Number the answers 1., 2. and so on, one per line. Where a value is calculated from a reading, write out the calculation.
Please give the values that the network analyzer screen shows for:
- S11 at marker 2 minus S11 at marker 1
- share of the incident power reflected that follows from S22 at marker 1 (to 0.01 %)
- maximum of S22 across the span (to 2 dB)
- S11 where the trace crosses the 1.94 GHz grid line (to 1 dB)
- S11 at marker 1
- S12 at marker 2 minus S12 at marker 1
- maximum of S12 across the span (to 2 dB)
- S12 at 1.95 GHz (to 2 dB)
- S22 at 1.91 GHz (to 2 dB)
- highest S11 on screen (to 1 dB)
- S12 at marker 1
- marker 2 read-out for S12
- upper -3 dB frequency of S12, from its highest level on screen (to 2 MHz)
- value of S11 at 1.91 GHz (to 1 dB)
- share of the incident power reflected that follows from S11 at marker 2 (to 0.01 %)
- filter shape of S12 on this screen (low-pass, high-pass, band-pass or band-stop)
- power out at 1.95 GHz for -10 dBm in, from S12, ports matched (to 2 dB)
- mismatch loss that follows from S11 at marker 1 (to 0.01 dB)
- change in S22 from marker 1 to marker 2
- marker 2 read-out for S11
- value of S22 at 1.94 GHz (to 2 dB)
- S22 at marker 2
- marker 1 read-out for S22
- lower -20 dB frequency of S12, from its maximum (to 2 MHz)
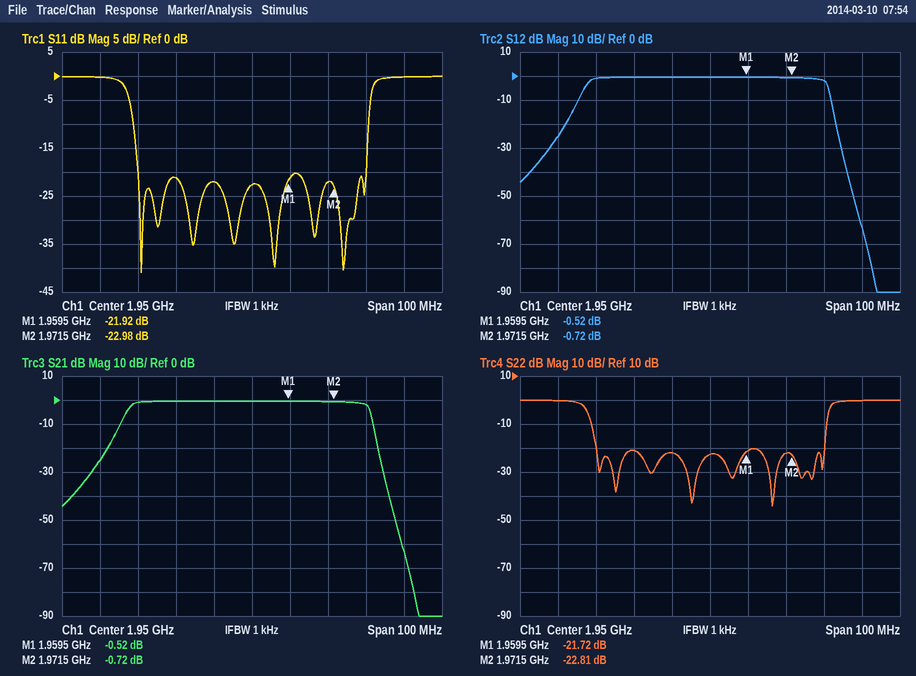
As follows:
1. -22.98 − (-21.92) = -1.06 dB
2. 10^(-21.72/10) ≈ 0.67 %
3. 0 dB
4. -22 dB
5. -21.92 dB
6. -0.72 − (-0.52) = -0.20 dB
7. 0 dB
8. 0 dB
9. 0 dB
10. 0 dB
11. -0.52 dB
12. -0.72 dB
13. 1.980 GHz
14. 0 dB
15. 10^(-22.98/10) ≈ 0.50 %
16. band-pass
17. -10 dBm + (0 dB) = -10 dBm
18. −10 log10(1 − 10^(-21.92/10)) ≈ 0.03 dB
19. -22.81 − (-21.72) = -1.09 dB
20. -22.98 dB
21. -22 dB
22. -22.81 dB
23. -21.72 dB
24. 1.912 GHz
